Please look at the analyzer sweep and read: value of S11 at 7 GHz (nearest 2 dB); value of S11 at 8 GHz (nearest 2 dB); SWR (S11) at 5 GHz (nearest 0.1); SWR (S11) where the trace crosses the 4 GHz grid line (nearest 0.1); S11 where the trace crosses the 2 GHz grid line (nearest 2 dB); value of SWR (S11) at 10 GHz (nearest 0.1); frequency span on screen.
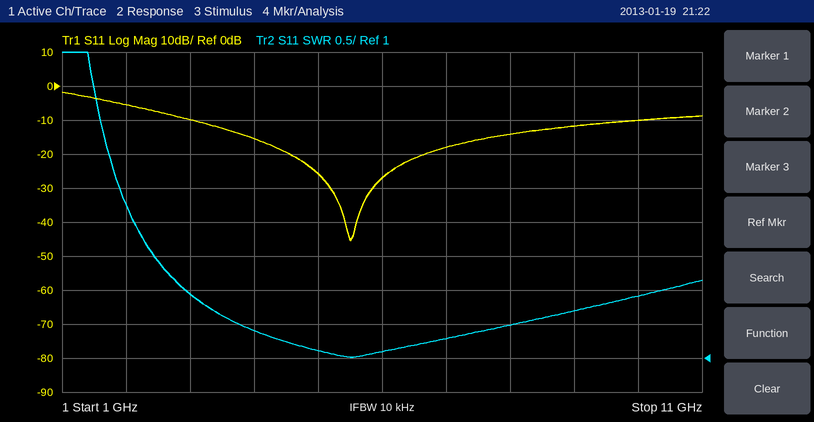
-18 dB
-14 dB
1.1
1.4
-6 dB
1.9
10 GHz
